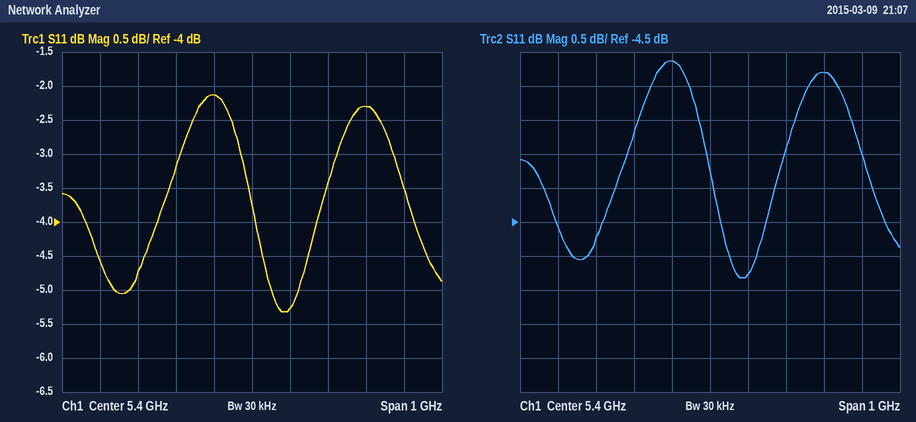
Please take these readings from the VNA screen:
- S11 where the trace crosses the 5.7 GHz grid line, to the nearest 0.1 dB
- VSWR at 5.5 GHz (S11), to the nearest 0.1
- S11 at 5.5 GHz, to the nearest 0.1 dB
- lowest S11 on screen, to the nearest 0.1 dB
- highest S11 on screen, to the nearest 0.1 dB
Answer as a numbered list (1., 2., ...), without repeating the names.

1. -2.3 dB
2. 3.4
3. -5.3 dB
4. -5.3 dB
5. -2.1 dB
